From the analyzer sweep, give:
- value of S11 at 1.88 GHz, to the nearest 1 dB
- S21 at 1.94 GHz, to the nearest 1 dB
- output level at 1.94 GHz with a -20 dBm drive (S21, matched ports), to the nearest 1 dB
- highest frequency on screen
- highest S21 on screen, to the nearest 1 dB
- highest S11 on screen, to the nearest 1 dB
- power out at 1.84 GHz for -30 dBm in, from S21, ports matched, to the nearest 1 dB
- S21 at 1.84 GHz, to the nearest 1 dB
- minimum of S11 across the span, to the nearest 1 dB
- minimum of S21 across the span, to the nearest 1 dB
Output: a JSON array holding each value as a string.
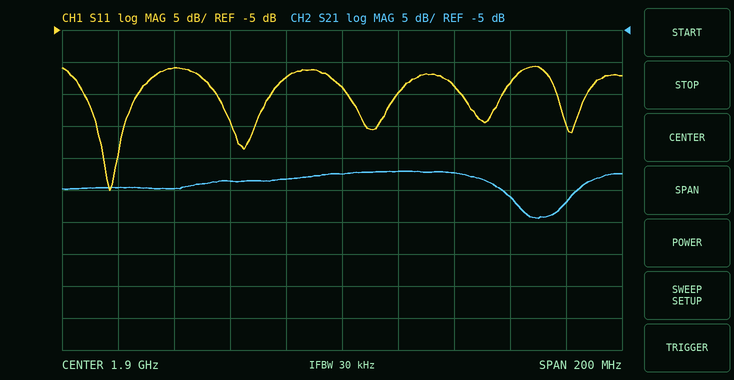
["-12 dB", "-27 dB", "-47 dBm", "2 GHz", "-27 dB", "-11 dB", "-60 dBm", "-30 dB", "-30 dB", "-34 dB"]
